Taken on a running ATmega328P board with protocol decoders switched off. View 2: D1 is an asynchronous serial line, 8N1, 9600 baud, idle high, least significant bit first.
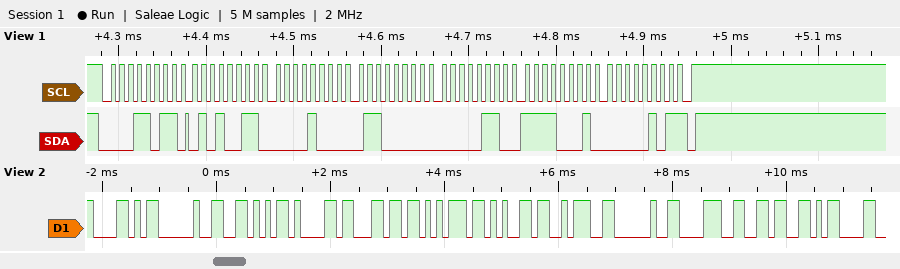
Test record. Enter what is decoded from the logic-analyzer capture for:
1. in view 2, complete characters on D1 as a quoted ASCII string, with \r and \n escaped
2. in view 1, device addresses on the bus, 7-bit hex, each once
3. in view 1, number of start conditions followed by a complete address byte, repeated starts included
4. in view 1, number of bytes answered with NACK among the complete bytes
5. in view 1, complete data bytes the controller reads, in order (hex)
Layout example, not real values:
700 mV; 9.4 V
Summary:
"X Value: 86\r"; 0x0D; 1; 1; 53 08 60 06 F1 05
